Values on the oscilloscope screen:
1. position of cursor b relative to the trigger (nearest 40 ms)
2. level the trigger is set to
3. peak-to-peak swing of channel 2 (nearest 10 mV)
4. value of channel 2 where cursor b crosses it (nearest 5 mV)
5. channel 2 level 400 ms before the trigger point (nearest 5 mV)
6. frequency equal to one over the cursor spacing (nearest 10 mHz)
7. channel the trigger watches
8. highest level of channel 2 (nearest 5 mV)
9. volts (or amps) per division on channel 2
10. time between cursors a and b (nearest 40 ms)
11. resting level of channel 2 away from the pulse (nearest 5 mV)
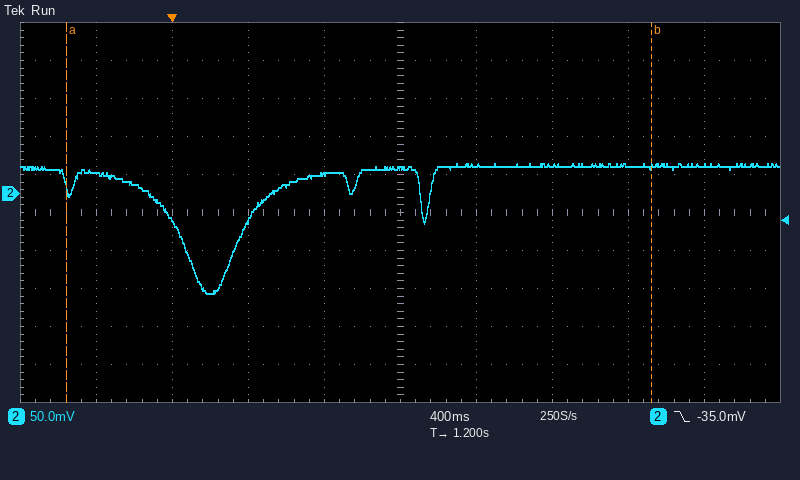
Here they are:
+2.52 s
-35.0 mV
170 mV
35 mV
25 mV
320 mHz
channel 2
40 mV
50 mV
3.08 s
35 mV
